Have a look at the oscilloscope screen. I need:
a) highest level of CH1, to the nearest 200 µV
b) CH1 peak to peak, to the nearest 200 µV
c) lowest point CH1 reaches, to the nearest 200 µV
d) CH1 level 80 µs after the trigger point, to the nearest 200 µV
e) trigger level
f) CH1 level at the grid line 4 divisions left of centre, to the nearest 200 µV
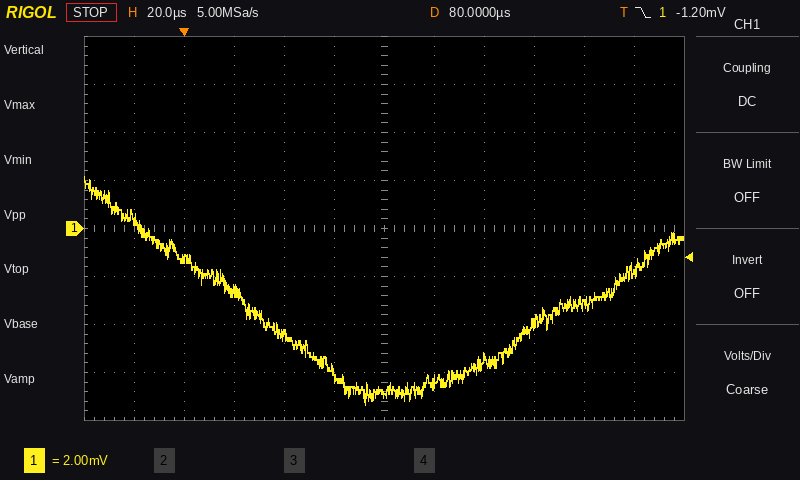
2.2 mV
9.6 mV
-7.4 mV
-6.8 mV
-1.20 mV
-1.2 mV
